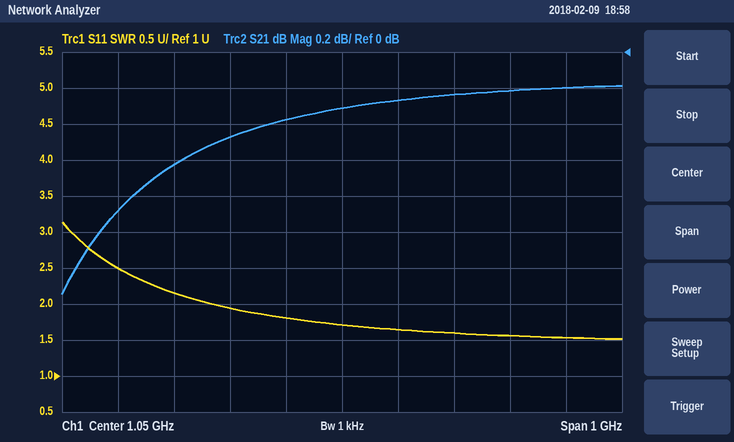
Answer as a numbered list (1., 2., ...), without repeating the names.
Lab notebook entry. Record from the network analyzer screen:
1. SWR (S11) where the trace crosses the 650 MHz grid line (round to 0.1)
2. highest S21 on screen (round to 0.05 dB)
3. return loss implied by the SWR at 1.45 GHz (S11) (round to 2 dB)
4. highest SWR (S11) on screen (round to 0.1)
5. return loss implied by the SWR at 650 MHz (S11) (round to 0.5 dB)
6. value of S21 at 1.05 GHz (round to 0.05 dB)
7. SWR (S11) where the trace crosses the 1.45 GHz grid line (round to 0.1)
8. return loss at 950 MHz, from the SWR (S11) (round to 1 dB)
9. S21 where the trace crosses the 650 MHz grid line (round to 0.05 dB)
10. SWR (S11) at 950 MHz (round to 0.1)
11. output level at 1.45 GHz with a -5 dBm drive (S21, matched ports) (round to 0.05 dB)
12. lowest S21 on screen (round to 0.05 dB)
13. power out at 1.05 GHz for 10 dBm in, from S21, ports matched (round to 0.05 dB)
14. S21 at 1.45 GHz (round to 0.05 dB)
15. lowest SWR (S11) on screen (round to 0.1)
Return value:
1. 2.5
2. -0.20 dB
3. 14 dB
4. 3.1
5. 7.5 dB
6. -0.30 dB
7. 1.5
8. 11 dB
9. -0.90 dB
10. 1.8
11. -5.20 dBm
12. -1.35 dB
13. 9.70 dBm
14. -0.20 dB
15. 1.5
